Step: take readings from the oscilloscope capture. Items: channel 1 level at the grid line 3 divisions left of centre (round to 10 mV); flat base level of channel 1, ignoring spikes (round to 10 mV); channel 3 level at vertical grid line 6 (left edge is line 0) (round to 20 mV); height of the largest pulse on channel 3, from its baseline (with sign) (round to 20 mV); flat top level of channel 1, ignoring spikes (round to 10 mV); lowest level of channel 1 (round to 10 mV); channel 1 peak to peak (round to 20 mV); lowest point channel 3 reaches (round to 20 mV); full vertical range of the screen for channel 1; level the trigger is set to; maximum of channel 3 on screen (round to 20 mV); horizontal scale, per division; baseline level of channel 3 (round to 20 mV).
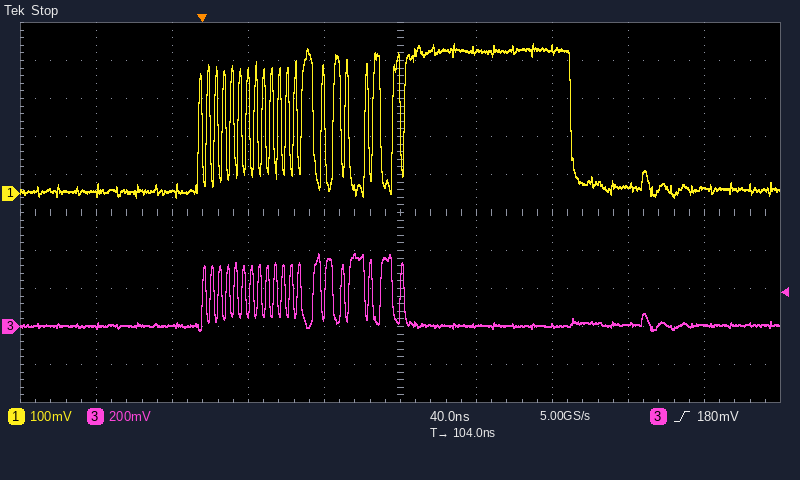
0 mV
10 mV
0 mV
+380 mV
380 mV
-10 mV
400 mV
-20 mV
1 V
180 mV
380 mV
40 ns
0 mV
